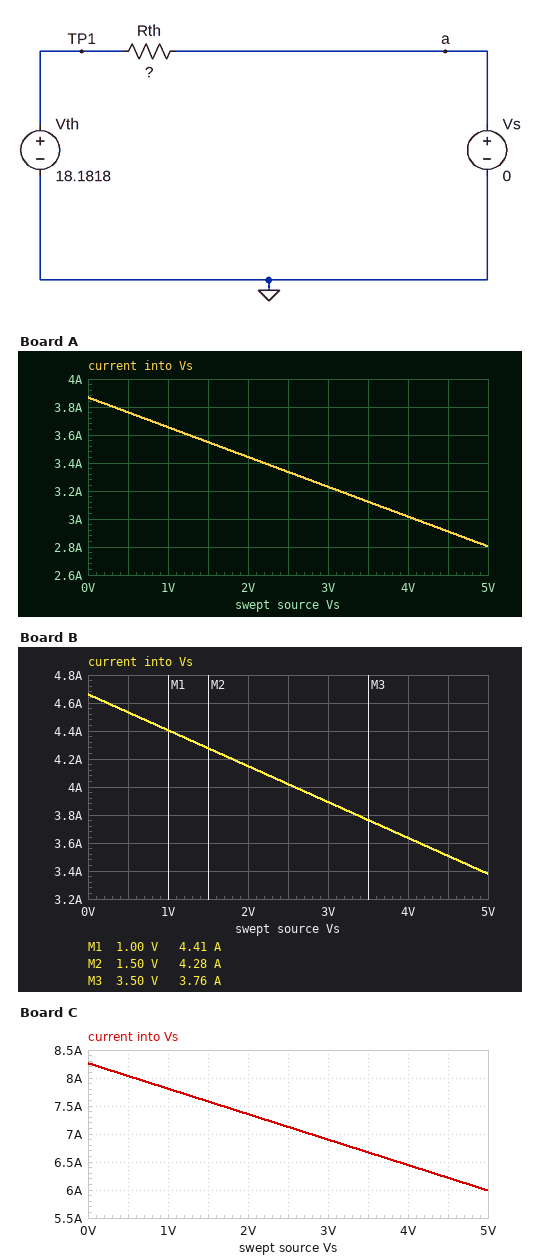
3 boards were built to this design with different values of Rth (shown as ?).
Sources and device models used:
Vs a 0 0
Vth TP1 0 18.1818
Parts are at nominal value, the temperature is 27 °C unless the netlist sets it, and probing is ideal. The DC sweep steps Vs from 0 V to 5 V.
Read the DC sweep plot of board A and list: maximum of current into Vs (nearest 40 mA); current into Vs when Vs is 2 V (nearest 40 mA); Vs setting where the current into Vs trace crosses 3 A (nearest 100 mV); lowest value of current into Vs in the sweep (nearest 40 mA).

3.88 A
3.44 A
4.1 V
2.80 A
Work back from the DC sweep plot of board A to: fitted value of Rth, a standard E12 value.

4.7 Ω
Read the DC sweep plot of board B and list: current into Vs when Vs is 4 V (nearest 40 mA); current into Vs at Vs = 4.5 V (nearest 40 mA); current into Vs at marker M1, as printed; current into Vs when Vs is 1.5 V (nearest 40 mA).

3.64 A
3.52 A
4.41 A
4.28 A
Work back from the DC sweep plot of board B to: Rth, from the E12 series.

3.9 Ω
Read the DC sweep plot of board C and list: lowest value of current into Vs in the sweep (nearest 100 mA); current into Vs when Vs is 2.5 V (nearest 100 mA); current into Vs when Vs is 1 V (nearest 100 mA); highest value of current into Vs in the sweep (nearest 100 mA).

6.0 A
7.1 A
7.8 A
8.3 A
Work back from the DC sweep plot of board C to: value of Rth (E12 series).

2.2 Ω
